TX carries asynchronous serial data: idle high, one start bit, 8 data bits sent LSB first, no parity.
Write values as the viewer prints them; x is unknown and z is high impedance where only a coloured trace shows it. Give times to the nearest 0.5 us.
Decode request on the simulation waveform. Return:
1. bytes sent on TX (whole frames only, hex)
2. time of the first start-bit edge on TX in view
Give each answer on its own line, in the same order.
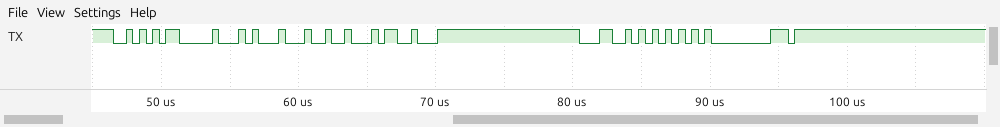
AA, 10, 11, 12, 13, 4C, 55, 00, FF
46.5 us
